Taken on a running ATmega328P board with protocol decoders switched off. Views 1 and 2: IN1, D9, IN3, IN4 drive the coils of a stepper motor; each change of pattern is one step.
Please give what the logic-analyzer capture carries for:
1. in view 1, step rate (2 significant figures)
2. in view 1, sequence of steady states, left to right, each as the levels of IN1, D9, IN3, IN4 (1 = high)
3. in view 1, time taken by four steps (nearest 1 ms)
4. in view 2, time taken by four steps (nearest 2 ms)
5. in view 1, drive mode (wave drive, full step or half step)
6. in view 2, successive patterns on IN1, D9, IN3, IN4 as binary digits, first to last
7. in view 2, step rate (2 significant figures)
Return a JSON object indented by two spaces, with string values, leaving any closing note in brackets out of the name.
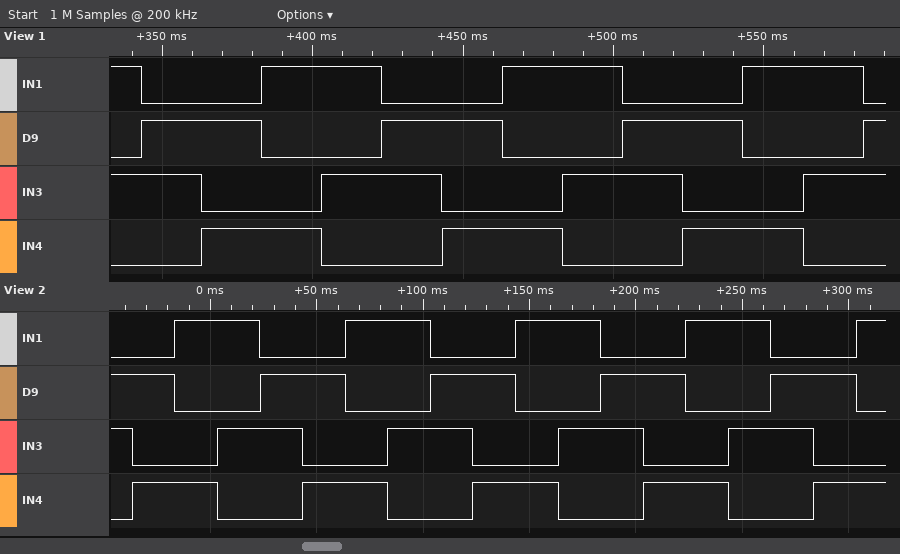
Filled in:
{
  "in view 1, step rate": "50 steps/s",
  "in view 1, sequence of steady states, left to right, each as the levels of IN1, D9, IN3, IN4": "1010 0110 0101 1001 1010 0110 0101 1001 1010 0110 0101 1001 1010 0110",
  "in view 1, time taken by four steps": "80 ms",
  "in view 2, time taken by four steps": "80 ms",
  "in view 1, drive mode": "full step",
  "in view 2, successive patterns on IN1, D9, IN3, IN4 as binary digits, first to last": "0110 0101 1001 1010 0110 0101 1001 1010 0110 0101 1001 1010 0110 0101 1001 1010 0110 0101 1001",
  "in view 2, step rate": "50 steps/s"
}
